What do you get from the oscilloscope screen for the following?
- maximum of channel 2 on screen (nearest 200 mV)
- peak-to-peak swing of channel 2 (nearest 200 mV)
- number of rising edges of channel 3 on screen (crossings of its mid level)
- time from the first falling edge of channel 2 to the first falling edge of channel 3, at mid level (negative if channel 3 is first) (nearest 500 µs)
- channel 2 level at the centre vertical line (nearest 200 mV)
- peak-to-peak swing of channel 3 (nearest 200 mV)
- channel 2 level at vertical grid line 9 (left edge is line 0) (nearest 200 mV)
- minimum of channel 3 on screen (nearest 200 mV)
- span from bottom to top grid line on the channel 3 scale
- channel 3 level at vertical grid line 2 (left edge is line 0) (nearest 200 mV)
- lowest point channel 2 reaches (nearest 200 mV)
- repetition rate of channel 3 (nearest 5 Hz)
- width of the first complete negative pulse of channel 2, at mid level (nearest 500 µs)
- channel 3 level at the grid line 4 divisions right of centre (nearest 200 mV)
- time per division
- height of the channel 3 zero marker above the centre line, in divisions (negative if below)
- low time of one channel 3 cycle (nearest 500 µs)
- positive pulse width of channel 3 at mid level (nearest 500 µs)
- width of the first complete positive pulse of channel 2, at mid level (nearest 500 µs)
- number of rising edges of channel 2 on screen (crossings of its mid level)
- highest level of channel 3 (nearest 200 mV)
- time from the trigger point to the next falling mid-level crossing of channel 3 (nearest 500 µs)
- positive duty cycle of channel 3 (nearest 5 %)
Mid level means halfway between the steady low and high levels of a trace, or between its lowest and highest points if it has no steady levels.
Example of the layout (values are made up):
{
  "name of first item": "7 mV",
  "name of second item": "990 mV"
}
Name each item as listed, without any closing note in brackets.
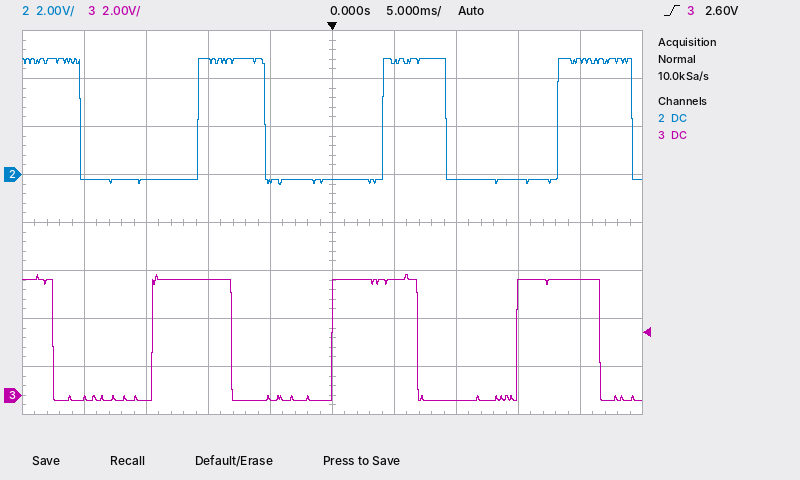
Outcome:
{
  "maximum of channel 2 on screen": "4.8 V",
  "peak-to-peak swing of channel 2": "5.2 V",
  "number of rising edges of channel 3 on screen": "3",
  "time from the first falling edge of channel 2 to the first falling edge of channel 3, at mid level (negative if channel 3 is first)": "-2.0 ms",
  "channel 2 level at the centre vertical line": "-200 mV",
  "peak-to-peak swing of channel 3": "5.2 V",
  "channel 2 level at vertical grid line 9 (left edge is line 0)": "4.8 V",
  "minimum of channel 3 on screen": "-200 mV",
  "span from bottom to top grid line on the channel 3 scale": "16 V",
  "channel 3 level at vertical grid line 2 (left edge is line 0)": "-200 mV",
  "lowest point channel 2 reaches": "-400 mV",
  "repetition rate of channel 3": "70 Hz",
  "width of the first complete negative pulse of channel 2, at mid level": "9.5 ms",
  "channel 3 level at the grid line 4 divisions right of centre": "4.8 V",
  "time per division": "5 ms",
  "height of the channel 3 zero marker above the centre line, in divisions": "-3.6 div",
  "low time of one channel 3 cycle": "8.0 ms",
  "positive pulse width of channel 3 at mid level": "6.5 ms",
  "width of the first complete positive pulse of channel 2, at mid level": "5.5 ms",
  "number of rising edges of channel 2 on screen": "3",
  "highest level of channel 3": "5.0 V",
  "time from the trigger point to the next falling mid-level crossing of channel 3": "7.0 ms",
  "positive duty cycle of channel 3": "45 %"
}
